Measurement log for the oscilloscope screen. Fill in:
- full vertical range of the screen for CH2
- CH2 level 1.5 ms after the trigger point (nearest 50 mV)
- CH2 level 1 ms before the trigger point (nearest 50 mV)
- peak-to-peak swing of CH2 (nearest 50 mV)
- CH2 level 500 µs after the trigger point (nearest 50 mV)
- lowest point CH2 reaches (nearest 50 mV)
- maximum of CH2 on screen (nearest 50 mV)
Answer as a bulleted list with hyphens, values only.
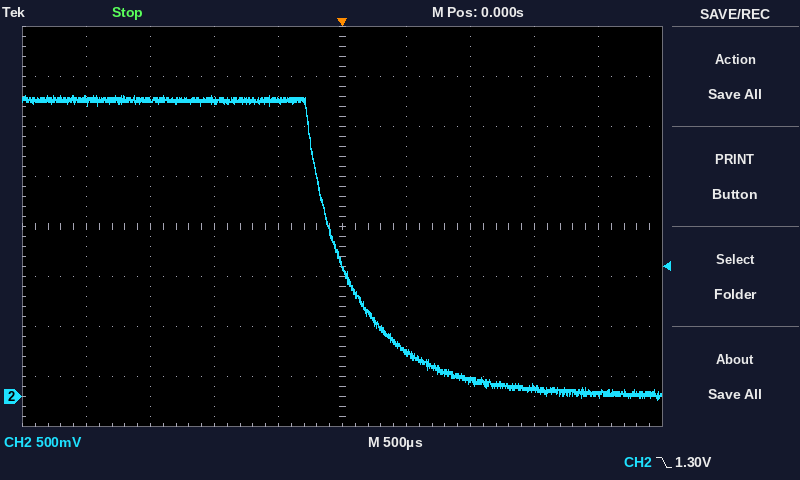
- 4 V
- 100 mV
- 2.95 V
- 3.05 V
- 450 mV
- -50 mV
- 3.00 V
